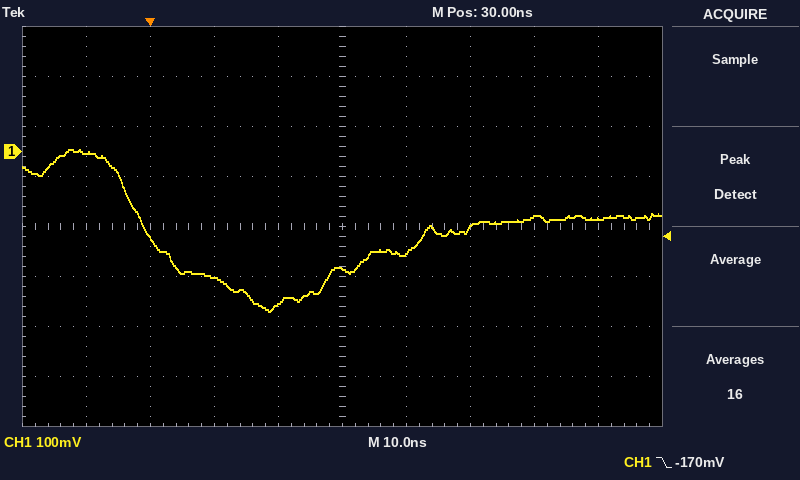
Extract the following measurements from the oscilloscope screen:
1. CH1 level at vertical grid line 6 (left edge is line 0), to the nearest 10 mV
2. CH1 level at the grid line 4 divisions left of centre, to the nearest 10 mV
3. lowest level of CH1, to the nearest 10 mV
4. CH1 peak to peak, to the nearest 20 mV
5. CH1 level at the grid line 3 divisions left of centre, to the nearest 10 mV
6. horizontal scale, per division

-200 mV
0 mV
-320 mV
320 mV
-170 mV
10 ns
